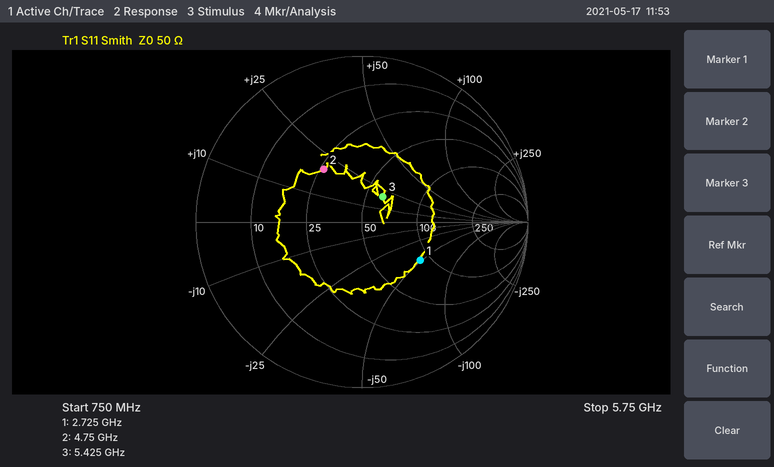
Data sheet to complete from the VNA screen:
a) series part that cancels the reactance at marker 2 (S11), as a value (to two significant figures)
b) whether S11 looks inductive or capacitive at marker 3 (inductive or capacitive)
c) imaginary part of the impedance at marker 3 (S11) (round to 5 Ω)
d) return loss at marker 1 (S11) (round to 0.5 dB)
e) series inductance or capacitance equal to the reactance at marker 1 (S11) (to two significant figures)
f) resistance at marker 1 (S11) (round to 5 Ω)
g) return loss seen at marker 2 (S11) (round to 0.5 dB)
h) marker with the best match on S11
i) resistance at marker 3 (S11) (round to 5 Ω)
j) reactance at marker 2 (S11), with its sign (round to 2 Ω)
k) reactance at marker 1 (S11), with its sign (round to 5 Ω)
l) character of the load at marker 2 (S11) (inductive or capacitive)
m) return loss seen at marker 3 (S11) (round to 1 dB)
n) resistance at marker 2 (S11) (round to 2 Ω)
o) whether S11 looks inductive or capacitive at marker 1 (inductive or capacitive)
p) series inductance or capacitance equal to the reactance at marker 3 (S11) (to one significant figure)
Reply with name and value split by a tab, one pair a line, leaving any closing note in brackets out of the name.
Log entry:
series part that cancels the reactance at marker 2 (S11), as a value	1.7 pF
whether S11 looks inductive or capacitive at marker 3	inductive
imaginary part of the impedance at marker 3 (S11)	+20 Ω
return loss at marker 1 (S11)	7.5 dB
series inductance or capacitance equal to the reactance at marker 1 (S11)	1.2 pF
resistance at marker 1 (S11)	85 Ω
return loss seen at marker 2 (S11)	8.0 dB
marker with the best match on S11	marker 3
resistance at marker 3 (S11)	60 Ω
reactance at marker 2 (S11), with its sign	+20 Ω
reactance at marker 1 (S11), with its sign	-50 Ω
character of the load at marker 2 (S11)	inductive
return loss seen at marker 3 (S11)	14 dB
resistance at marker 2 (S11)	26 Ω
whether S11 looks inductive or capacitive at marker 1	capacitive
series inductance or capacitance equal to the reactance at marker 3 (S11)	600 pH
